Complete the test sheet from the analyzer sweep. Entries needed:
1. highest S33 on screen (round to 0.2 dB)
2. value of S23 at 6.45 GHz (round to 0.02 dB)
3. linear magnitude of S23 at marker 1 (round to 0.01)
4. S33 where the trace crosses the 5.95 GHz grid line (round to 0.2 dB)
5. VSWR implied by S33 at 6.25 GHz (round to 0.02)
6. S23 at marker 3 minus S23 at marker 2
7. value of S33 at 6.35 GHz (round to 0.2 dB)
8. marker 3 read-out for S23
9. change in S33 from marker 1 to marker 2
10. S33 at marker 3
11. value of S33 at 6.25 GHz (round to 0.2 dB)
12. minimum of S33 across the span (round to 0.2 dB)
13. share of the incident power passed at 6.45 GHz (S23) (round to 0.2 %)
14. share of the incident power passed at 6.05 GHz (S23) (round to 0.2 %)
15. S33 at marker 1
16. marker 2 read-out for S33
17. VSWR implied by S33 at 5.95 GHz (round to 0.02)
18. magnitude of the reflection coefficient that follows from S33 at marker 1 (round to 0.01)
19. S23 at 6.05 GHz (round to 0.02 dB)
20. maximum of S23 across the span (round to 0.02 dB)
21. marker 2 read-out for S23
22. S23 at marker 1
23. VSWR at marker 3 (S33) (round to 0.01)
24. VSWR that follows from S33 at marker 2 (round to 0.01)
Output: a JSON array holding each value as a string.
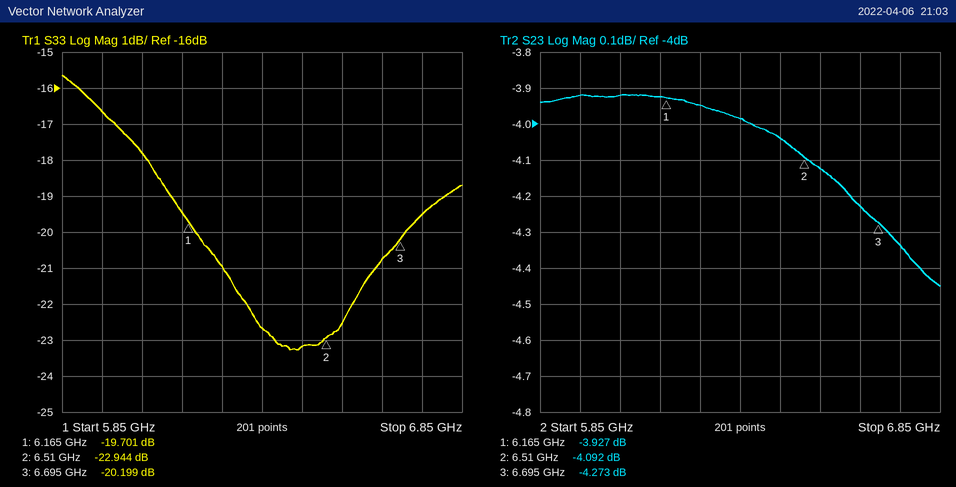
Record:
["-15.6 dB", "-4.04 dB", "0.64", "-16.6 dB", "1.20", "-0.181 dB", "-22.6 dB", "-4.273 dB", "-3.243 dB", "-20.199 dB", "-21.0 dB", "-23.2 dB", "39.4 %", "40.6 %", "-19.701 dB", "-22.944 dB", "1.34", "0.10", "-3.92 dB", "-3.92 dB", "-4.092 dB", "-3.927 dB", "1.22", "1.15"]
